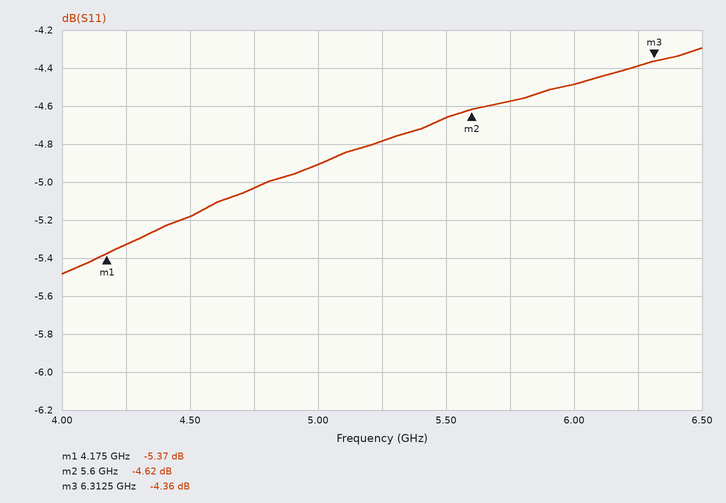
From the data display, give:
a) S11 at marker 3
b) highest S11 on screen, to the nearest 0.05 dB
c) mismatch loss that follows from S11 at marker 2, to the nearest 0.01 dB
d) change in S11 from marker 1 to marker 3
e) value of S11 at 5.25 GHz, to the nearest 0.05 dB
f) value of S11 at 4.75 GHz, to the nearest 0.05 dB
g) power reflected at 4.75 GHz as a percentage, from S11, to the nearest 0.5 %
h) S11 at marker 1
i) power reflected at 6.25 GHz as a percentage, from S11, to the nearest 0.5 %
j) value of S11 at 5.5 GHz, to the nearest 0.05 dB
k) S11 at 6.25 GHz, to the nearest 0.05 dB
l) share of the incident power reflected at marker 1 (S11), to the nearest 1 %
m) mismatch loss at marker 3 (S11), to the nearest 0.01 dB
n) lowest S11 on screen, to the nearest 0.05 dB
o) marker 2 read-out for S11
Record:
-4.36 dB
-4.30 dB
1.84 dB
1.01 dB
-4.80 dB
-5.05 dB
31.5 %
-5.37 dB
36.5 %
-4.65 dB
-4.40 dB
29 %
1.98 dB
-5.50 dB
-4.62 dB
